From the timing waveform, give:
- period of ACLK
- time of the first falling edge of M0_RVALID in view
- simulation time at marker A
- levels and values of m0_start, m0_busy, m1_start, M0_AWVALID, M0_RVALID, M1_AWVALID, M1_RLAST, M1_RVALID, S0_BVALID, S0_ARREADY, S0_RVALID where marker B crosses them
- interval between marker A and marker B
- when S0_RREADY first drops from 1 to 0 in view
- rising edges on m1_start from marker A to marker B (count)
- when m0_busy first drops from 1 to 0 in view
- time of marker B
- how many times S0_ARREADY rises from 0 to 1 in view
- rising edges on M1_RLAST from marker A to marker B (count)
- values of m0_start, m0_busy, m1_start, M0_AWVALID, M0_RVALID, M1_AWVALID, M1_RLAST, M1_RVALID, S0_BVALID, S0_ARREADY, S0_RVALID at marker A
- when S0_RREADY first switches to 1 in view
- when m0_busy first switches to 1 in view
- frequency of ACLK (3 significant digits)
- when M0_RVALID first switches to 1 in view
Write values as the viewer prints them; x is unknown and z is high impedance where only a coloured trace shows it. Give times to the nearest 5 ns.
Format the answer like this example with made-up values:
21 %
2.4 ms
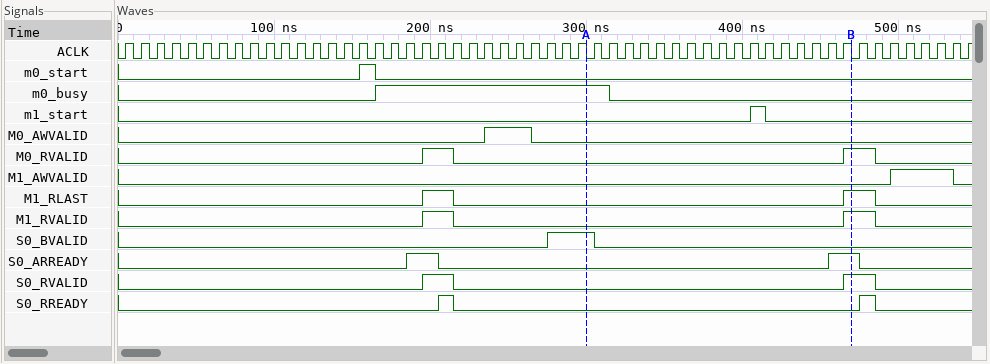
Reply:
10 ns
215 ns
300 ns
m0_start=0, m0_busy=0, m1_start=0, M0_AWVALID=0, M0_RVALID=1, M1_AWVALID=0, M1_RLAST=1, M1_RVALID=1, S0_BVALID=0, S0_ARREADY=1, S0_RVALID=1
170 ns
215 ns
1
315 ns
470 ns
2
1
m0_start=0, m0_busy=1, m1_start=0, M0_AWVALID=0, M0_RVALID=0, M1_AWVALID=0, M1_RLAST=0, M1_RVALID=0, S0_BVALID=1, S0_ARREADY=0, S0_RVALID=0
205 ns
165 ns
100 MHz
195 ns
